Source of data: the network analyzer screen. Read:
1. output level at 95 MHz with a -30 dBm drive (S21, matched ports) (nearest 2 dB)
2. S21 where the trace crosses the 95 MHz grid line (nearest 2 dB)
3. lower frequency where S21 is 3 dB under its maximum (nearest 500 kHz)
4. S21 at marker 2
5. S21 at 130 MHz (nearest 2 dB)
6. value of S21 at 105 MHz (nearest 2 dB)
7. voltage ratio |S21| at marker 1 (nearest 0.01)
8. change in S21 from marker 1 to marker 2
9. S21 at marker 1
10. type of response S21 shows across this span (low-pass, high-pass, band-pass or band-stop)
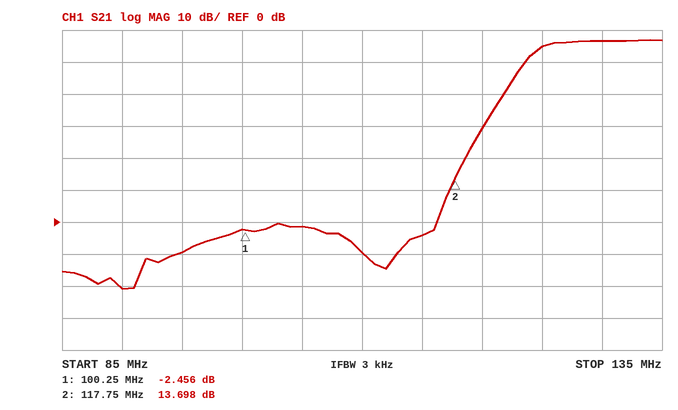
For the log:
-40 dBm
-10 dB
124.5 MHz
13.698 dB
56 dB
-2 dB
0.75
16.154 dB
-2.456 dB
high-pass
